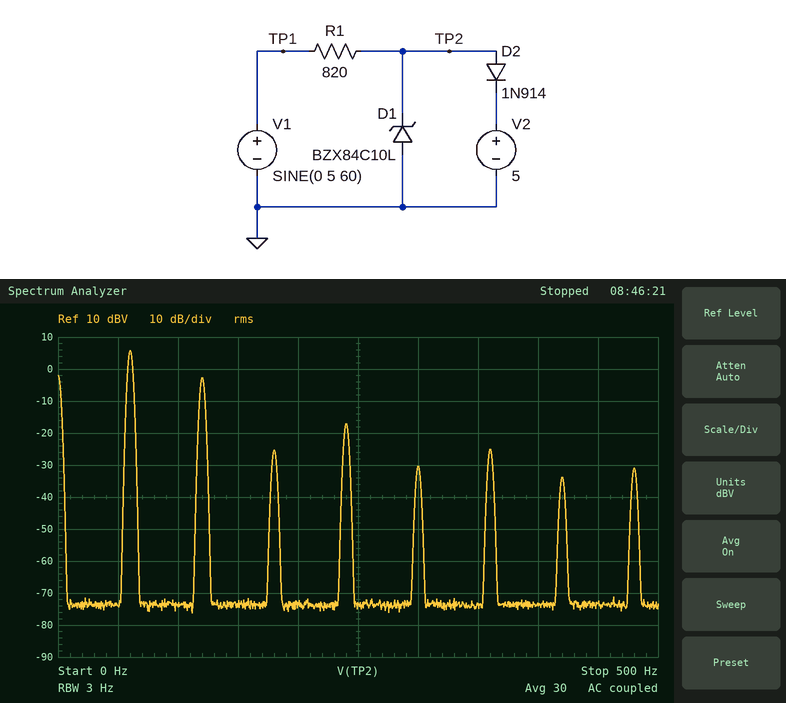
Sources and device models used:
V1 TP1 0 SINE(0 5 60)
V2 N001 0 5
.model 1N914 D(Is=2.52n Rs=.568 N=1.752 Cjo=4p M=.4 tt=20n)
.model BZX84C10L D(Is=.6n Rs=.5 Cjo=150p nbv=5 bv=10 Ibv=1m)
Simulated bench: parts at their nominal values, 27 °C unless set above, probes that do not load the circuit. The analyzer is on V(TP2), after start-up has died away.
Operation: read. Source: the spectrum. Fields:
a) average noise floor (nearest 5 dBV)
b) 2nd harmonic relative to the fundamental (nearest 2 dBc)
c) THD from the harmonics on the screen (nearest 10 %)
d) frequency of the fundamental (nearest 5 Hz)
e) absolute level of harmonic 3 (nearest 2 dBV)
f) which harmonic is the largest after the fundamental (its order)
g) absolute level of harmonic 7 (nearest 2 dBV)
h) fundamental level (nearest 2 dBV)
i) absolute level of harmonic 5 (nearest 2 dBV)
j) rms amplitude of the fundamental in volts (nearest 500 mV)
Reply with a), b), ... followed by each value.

a) -75 dBV
b) -8 dBc
c) 40 %
d) 60 Hz
e) -26 dBV
f) 2
g) -34 dBV
h) 6 dBV
i) -30 dBV
j) 2.0 V
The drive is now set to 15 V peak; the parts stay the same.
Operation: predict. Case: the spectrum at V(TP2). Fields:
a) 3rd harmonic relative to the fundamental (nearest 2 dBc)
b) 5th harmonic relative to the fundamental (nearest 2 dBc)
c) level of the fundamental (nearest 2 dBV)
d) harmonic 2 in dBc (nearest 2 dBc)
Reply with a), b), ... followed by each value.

a) -12 dBc
b) -20 dBc
c) 8 dBV
d) -16 dBc
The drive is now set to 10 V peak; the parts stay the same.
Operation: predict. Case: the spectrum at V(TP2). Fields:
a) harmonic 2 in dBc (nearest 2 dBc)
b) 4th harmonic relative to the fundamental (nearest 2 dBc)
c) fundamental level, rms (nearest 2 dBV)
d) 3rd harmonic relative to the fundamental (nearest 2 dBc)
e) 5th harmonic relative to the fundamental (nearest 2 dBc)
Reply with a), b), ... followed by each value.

a) -12 dBc
b) -16 dBc
c) 8 dBV
d) -14 dBc
e) -30 dBc
